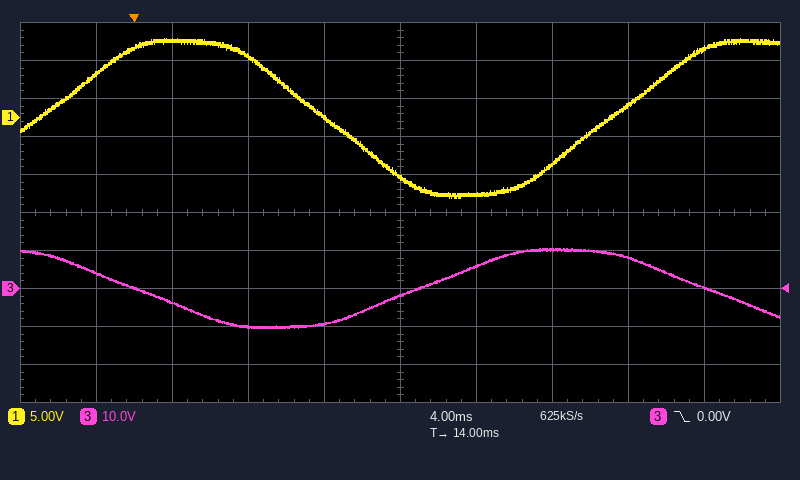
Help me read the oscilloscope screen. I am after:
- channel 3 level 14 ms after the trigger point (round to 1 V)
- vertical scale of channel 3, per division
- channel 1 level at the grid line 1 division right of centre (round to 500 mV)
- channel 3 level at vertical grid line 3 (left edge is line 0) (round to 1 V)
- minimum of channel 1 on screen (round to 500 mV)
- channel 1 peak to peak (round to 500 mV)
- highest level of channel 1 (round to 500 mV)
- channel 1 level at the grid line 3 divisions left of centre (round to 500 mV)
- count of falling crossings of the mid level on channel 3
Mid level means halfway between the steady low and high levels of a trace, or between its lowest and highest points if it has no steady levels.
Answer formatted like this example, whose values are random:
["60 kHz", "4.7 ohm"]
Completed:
["-2 V", "10 V", "-10.0 V", "-10 V", "-10.5 V", "21.0 V", "10.5 V", "10.0 V", "2"]
